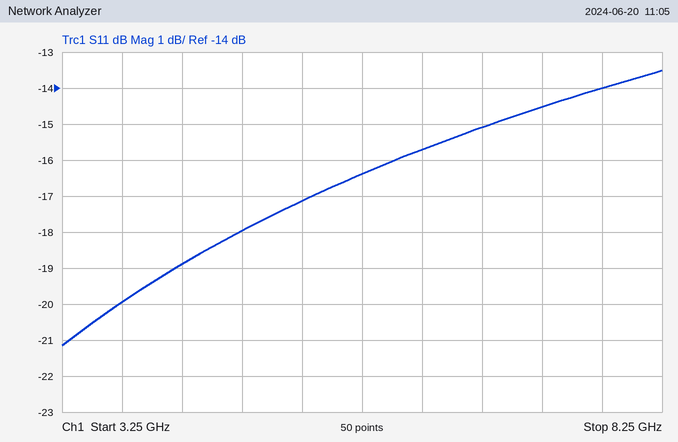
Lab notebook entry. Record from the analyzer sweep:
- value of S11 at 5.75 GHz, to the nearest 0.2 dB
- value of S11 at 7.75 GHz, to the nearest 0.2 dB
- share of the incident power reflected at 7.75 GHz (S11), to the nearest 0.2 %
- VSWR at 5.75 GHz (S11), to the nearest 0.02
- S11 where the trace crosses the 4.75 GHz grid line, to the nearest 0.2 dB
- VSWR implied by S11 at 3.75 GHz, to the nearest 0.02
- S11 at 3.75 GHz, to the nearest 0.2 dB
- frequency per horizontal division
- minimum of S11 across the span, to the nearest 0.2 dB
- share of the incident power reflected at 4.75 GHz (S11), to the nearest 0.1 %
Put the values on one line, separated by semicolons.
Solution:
-16.4 dB; -14.0 dB; 4.0 %; 1.36; -18.0 dB; 1.22; -20.0 dB; 500 MHz; -21.2 dB; 1.6 %
